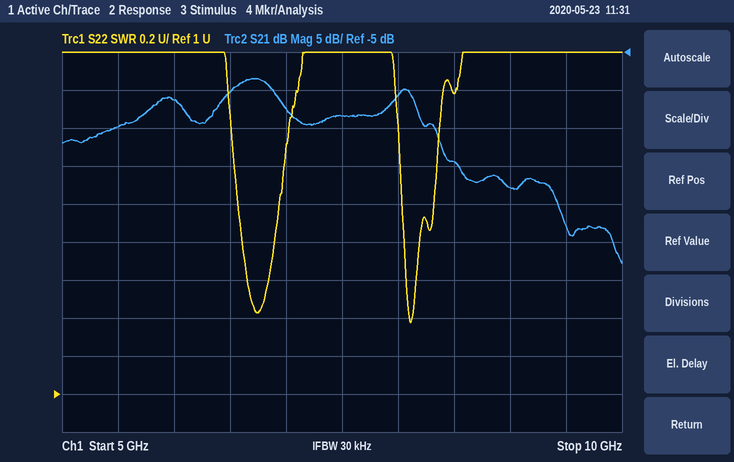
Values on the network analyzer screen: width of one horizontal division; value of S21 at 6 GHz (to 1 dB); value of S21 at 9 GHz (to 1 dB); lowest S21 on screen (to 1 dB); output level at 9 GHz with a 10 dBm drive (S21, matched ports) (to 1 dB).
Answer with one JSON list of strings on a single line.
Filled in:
["500 MHz", "-11 dB", "-23 dB", "-33 dB", "-13 dBm"]
